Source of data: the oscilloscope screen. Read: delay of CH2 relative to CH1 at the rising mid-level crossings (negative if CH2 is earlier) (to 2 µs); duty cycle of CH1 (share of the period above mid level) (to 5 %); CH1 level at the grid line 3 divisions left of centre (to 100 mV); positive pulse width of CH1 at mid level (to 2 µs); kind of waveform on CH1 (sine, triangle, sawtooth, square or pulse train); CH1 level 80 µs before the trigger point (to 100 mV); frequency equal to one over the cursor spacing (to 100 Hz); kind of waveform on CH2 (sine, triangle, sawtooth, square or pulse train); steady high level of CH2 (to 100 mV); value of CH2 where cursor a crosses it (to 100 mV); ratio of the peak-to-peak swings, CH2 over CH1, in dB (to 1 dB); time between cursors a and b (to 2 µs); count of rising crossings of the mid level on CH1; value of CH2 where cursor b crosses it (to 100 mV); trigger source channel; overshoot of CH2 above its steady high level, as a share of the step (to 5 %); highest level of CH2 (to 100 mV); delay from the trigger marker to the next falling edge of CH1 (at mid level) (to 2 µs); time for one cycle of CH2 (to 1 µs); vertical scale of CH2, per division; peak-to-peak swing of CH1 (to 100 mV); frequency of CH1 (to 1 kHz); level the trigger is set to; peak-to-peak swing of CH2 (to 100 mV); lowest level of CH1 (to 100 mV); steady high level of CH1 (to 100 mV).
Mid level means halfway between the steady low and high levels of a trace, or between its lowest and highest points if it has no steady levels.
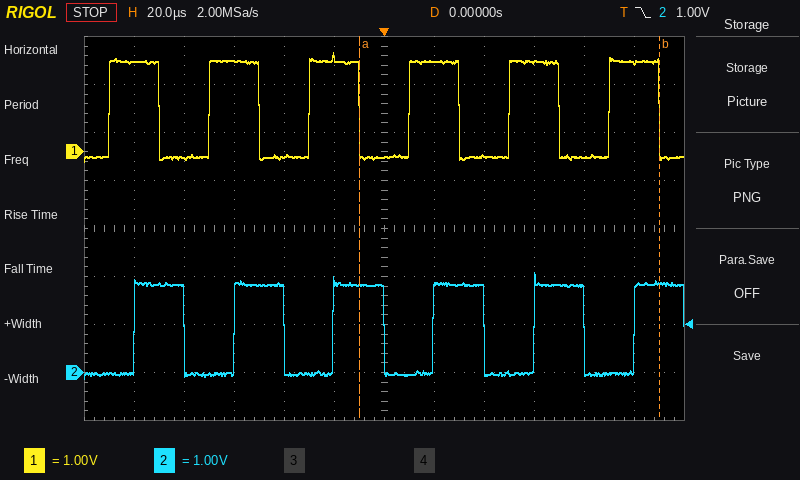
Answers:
+10 µs
50 %
1.9 V
20 µs
square
-100 mV
8.3 kHz
square
1.8 V
1.8 V
0 dB
120 µs
6
1.9 V
CH2
15 %
2.1 V
30 µs
40 µs
1 V
2.3 V
25 kHz
1.00 V
2.2 V
-200 mV
1.9 V
